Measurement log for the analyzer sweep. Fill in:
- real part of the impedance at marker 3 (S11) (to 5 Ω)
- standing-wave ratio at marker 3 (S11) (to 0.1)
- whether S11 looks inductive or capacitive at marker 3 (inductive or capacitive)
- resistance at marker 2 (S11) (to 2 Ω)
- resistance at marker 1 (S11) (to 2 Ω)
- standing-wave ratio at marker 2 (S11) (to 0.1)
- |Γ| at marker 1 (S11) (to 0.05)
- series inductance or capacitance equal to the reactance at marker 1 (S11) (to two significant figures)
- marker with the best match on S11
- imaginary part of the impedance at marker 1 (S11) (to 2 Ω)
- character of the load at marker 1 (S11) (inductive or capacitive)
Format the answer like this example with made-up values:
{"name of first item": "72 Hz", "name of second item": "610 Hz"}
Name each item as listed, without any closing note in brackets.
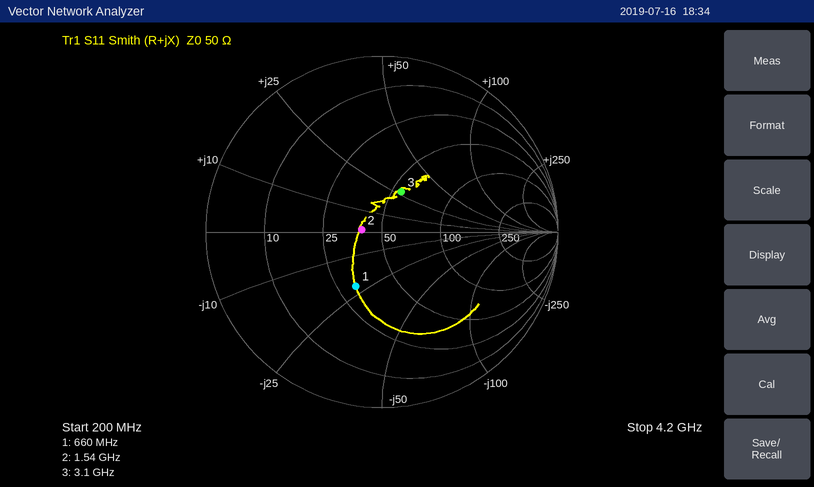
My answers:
{"real part of the impedance at marker 3 (S11)": "55 Ω", "standing-wave ratio at marker 3 (S11)": "1.7", "whether S11 looks inductive or capacitive at marker 3": "inductive", "resistance at marker 2 (S11)": "40 Ω", "resistance at marker 1 (S11)": "32 Ω", "standing-wave ratio at marker 2 (S11)": "1.3", "|Γ| at marker 1 (S11)": "0.35", "series inductance or capacitance equal to the reactance at marker 1 (S11)": "11 pF", "marker with the best match on S11": "marker 2", "imaginary part of the impedance at marker 1 (S11)": "-22 Ω", "character of the load at marker 1 (S11)": "capacitive"}
